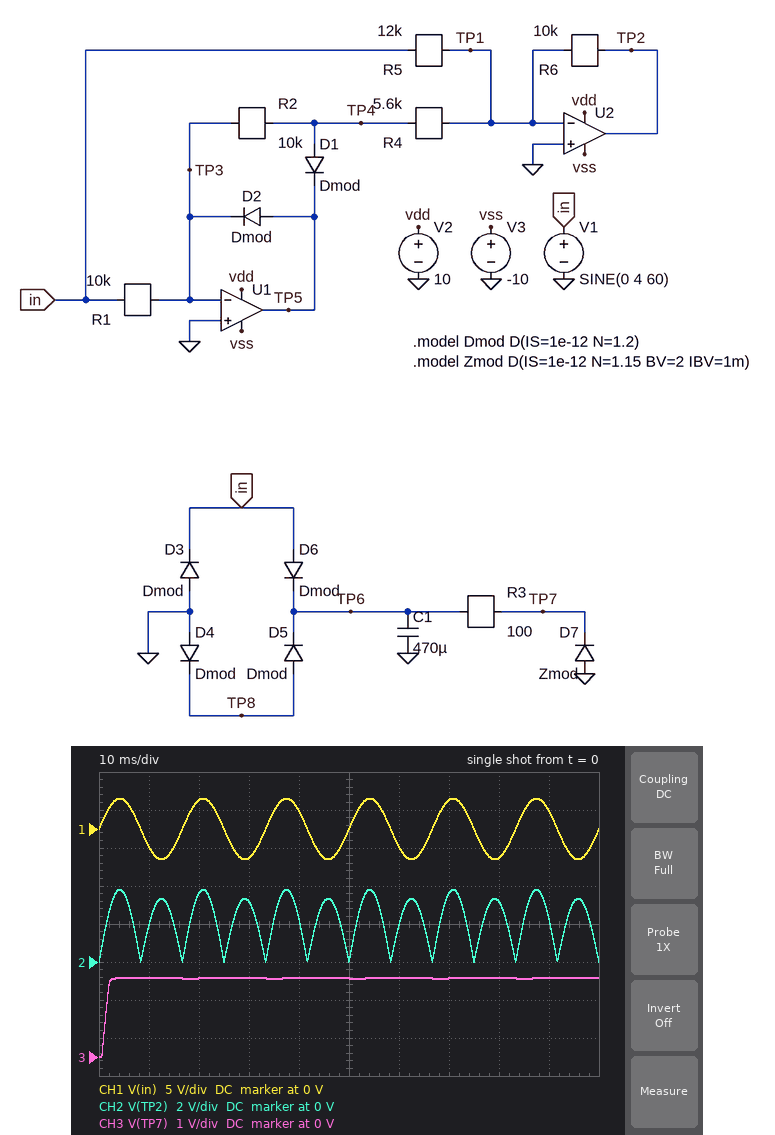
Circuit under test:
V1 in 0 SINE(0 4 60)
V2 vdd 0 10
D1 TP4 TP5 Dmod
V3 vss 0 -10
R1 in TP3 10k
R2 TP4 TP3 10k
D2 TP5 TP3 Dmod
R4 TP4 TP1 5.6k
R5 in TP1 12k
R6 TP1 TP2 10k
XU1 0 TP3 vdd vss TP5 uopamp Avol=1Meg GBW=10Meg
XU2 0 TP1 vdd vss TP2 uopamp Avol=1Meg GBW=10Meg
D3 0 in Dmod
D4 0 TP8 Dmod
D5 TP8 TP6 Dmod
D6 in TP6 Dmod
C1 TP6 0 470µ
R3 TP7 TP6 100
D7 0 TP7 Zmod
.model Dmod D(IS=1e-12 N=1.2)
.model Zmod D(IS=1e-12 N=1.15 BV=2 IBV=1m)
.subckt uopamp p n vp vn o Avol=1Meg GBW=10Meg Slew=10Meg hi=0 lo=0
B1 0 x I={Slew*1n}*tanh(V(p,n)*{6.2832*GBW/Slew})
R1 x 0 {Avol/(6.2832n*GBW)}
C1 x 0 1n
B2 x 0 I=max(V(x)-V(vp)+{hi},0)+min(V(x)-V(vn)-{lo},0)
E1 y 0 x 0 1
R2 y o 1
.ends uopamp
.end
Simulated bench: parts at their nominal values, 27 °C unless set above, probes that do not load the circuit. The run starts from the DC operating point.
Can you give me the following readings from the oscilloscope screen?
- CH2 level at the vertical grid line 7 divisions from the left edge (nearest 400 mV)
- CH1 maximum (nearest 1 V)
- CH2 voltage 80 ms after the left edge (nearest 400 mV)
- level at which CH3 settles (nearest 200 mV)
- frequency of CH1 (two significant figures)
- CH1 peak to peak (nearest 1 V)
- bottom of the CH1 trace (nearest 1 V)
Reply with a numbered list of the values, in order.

1. 3.6 V
2. 4 V
3. 3.2 V
4. 2.0 V
5. 60 Hz
6. 8 V
7. -4 V
